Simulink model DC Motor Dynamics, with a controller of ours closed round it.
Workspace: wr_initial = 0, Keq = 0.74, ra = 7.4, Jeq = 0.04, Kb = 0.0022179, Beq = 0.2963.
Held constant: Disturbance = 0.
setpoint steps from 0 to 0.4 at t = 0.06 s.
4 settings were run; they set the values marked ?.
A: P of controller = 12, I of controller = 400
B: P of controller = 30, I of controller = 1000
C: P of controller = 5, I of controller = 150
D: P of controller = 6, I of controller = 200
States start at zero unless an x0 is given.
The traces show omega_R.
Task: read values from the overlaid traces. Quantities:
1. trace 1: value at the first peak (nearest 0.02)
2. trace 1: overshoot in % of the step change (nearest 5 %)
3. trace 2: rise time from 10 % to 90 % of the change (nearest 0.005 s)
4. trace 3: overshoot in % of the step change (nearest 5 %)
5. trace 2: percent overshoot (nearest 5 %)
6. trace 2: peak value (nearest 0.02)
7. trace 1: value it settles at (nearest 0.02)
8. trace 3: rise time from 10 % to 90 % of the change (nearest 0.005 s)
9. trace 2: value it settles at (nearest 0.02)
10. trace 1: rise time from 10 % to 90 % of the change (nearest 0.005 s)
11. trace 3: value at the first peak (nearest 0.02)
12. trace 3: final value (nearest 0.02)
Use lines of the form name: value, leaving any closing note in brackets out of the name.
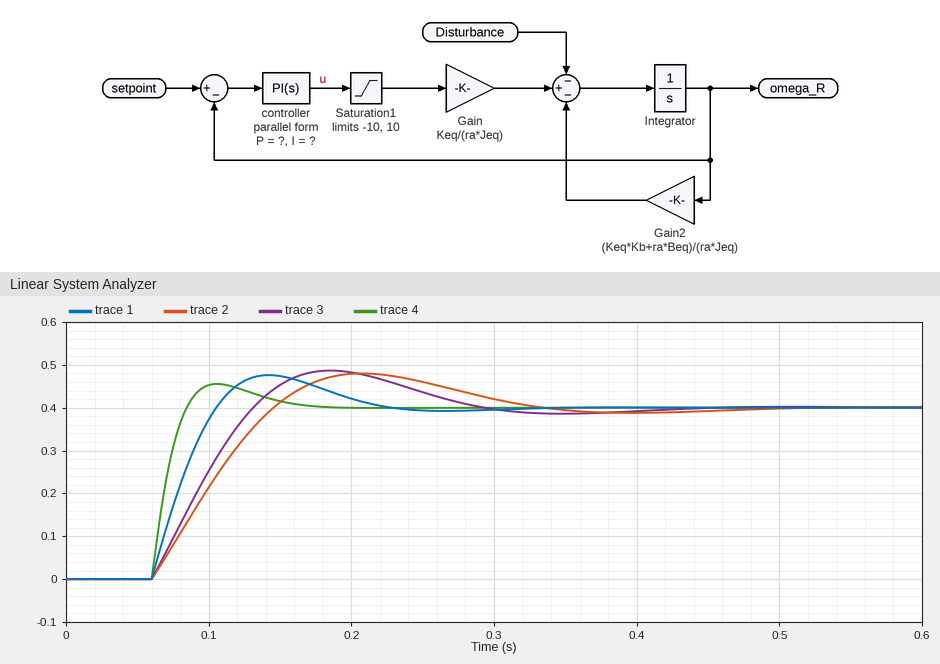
trace 1: value at the first peak: 0.48
trace 1: overshoot in % of the step change: 20 %
trace 2: rise time from 10 % to 90 % of the change: 0.065 s
trace 3: overshoot in % of the step change: 20 %
trace 2: percent overshoot: 20 %
trace 2: peak value: 0.48
trace 1: value it settles at: 0.40
trace 3: rise time from 10 % to 90 % of the change: 0.055 s
trace 2: value it settles at: 0.40
trace 1: rise time from 10 % to 90 % of the change: 0.035 s
trace 3: value at the first peak: 0.48
trace 3: final value: 0.40
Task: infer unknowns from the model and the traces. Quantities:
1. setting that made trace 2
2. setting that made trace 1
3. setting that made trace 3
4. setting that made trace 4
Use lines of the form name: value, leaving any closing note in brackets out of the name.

setting that made trace 2: C
setting that made trace 1: A
setting that made trace 3: D
setting that made trace 4: B
